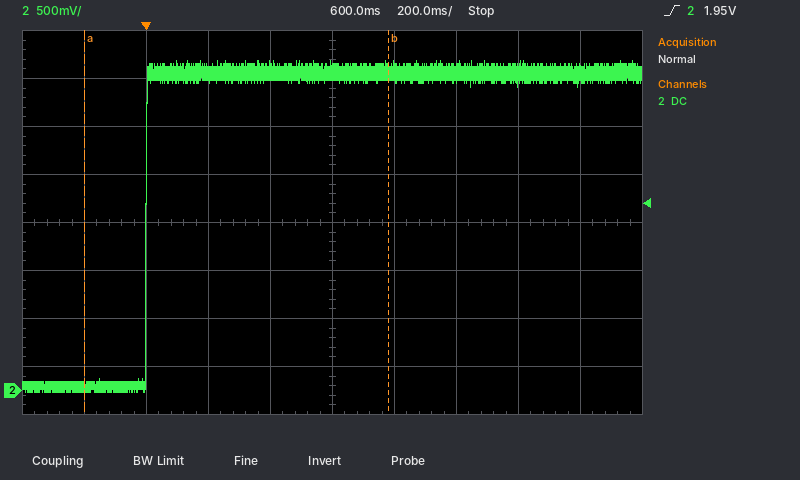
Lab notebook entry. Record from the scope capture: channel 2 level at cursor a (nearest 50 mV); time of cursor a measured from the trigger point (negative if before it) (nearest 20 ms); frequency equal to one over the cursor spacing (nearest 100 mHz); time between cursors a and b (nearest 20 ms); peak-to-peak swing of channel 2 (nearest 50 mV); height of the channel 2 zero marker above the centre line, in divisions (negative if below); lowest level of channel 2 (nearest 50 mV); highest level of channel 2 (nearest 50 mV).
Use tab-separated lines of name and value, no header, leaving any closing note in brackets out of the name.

channel 2 level at cursor a	50 mV
time of cursor a measured from the trigger point (negative if before it)	-200 ms
frequency equal to one over the cursor spacing	1.0 Hz
time between cursors a and b	980 ms
peak-to-peak swing of channel 2	3.45 V
height of the channel 2 zero marker above the centre line, in divisions	-3.5 div
lowest level of channel 2	0 mV
highest level of channel 2	3.45 V
